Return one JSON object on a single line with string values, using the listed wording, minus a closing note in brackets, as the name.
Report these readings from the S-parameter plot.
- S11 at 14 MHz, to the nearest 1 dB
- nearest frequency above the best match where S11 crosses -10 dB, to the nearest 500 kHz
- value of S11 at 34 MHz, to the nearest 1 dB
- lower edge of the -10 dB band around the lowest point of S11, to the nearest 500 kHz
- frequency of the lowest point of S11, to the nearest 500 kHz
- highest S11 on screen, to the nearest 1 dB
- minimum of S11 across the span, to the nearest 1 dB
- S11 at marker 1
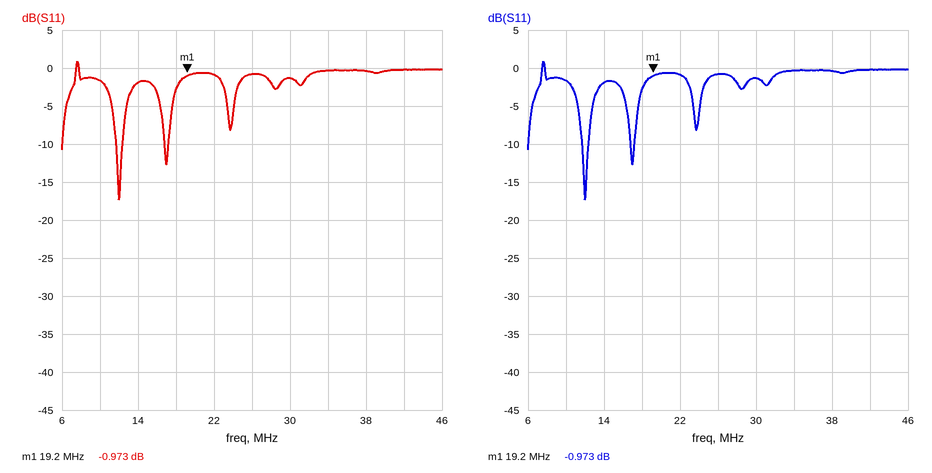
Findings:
{"S11 at 14 MHz, to the nearest 1 dB": "-2 dB", "nearest frequency above the best match where S11 crosses -10 dB, to the nearest 500 kHz": "12.5 MHz", "value of S11 at 34 MHz, to the nearest 1 dB": "0 dB", "lower edge of the -10 dB band around the lowest point of S11, to the nearest 500 kHz": "11.5 MHz", "frequency of the lowest point of S11, to the nearest 500 kHz": "12.0 MHz", "highest S11 on screen, to the nearest 1 dB": "1 dB", "minimum of S11 across the span, to the nearest 1 dB": "-17 dB", "S11 at marker 1": "-0.973 dB"}
